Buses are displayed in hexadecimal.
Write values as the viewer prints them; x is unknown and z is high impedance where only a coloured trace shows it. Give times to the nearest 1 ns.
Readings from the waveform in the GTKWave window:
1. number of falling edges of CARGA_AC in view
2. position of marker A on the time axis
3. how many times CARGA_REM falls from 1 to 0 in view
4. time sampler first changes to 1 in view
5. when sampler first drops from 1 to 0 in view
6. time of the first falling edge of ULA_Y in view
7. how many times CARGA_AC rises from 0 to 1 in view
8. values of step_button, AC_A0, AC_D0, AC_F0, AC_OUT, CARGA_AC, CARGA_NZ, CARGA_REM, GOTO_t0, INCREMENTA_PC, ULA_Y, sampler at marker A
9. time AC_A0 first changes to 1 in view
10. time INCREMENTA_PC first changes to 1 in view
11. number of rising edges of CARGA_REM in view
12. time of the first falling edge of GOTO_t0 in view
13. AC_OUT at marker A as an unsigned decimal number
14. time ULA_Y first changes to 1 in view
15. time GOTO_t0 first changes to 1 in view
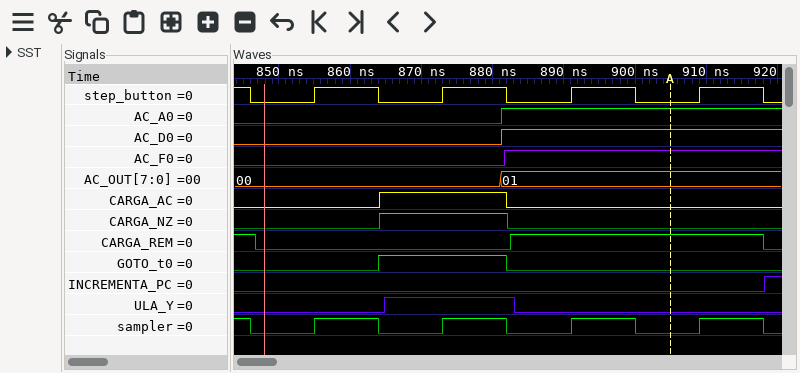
1
905 ns
2
855 ns
846 ns
883 ns
1
step_button=0, AC_A0=1, AC_D0=1, AC_F0=1, AC_OUT=01, CARGA_AC=0, CARGA_NZ=0, CARGA_REM=1, GOTO_t0=0, INCREMENTA_PC=0, ULA_Y=0, sampler=0
881 ns
918 ns
1
882 ns
1
865 ns
864 ns
